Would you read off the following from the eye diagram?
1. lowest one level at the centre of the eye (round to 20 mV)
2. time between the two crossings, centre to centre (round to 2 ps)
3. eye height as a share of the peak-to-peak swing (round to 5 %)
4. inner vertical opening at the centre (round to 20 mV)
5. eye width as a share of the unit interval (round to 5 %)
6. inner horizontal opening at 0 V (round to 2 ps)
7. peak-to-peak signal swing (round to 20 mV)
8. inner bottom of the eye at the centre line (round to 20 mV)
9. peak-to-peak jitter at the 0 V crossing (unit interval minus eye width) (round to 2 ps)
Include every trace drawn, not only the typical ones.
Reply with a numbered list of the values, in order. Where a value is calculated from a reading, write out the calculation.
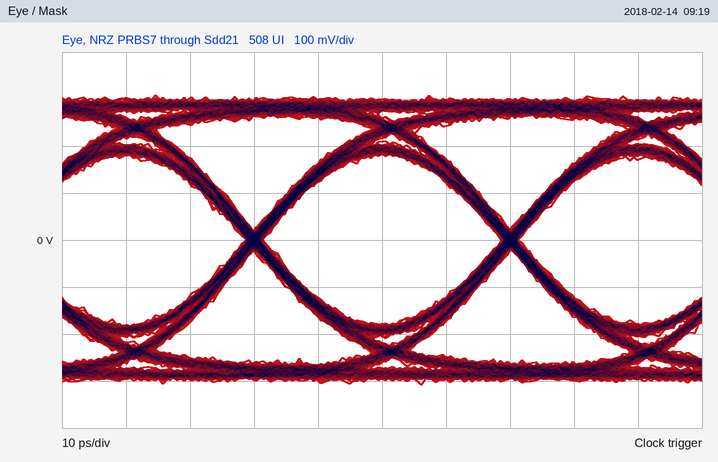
1. 180 mV
2. 40 ps
3. 360 mV / 620 mV ≈ 58.1 %, so 60 % to the nearest 5 %
4. 360 mV
5. 38 ps / 40 ps ≈ 95 %
6. 38 ps
7. 620 mV
8. -180 mV
9. 2 ps
